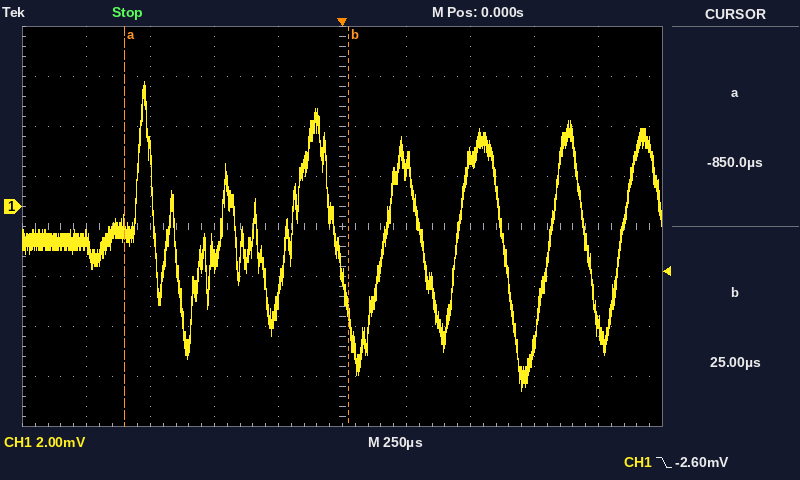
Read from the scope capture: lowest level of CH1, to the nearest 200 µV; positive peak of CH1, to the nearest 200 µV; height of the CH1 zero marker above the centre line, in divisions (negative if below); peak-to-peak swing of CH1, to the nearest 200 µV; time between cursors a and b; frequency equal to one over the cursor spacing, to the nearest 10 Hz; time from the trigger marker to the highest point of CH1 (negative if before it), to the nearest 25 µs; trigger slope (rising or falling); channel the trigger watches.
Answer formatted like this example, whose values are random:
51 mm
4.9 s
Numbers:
-7.4 mV
5.0 mV
+0.4 div
12.4 mV
875 µs
1.14 kHz
-775 µs
falling
CH1
